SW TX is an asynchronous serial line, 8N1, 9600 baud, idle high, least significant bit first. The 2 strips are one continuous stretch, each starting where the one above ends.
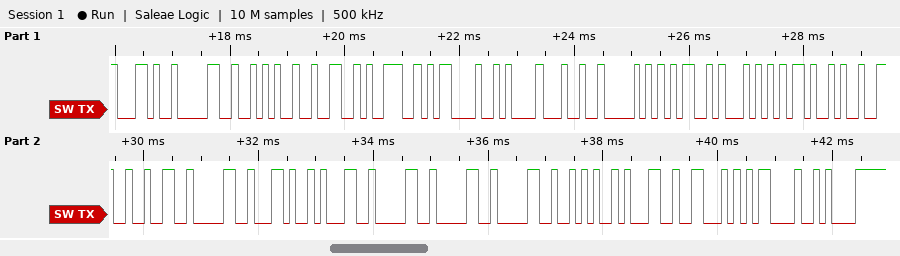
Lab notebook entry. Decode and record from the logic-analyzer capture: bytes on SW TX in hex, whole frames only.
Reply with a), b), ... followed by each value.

a) 0x2C 0x30 0x2A 0x32 0x39 0x0D 0x0A 0x24 0x50 0x4D 0x54 0x4B 0x32 0x32 0x30 0x2C 0x31 0x30 0x30 0x30 0x2A 0x31 0x46 0x0D 0x0A
